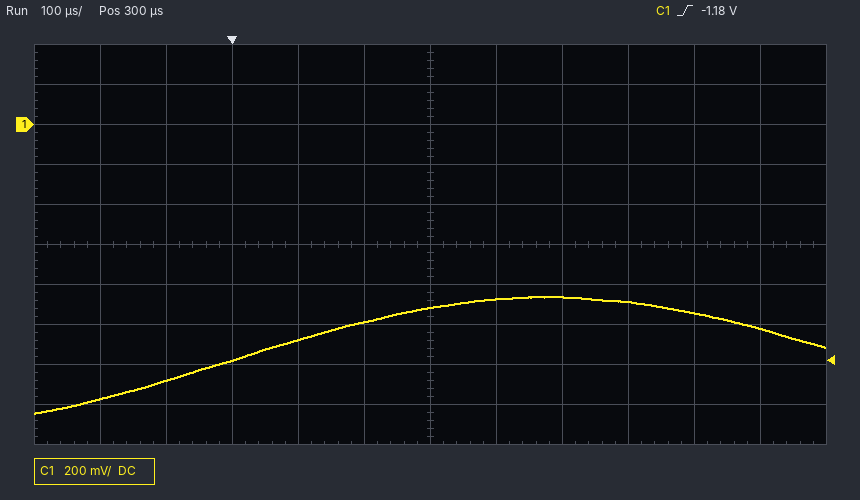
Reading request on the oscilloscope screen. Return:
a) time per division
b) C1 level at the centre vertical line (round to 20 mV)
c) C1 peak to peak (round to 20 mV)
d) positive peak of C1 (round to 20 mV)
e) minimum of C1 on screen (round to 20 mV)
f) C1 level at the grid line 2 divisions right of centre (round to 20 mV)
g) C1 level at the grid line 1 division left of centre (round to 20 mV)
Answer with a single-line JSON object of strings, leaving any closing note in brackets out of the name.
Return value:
{"time per division": "100 µs", "C1 level at the centre vertical line": "-920 mV", "C1 peak to peak": "580 mV", "positive peak of C1": "-860 mV", "minimum of C1 on screen": "-1.44 V", "C1 level at the grid line 2 divisions right of centre": "-860 mV", "C1 level at the grid line 1 division left of centre": "-980 mV"}
